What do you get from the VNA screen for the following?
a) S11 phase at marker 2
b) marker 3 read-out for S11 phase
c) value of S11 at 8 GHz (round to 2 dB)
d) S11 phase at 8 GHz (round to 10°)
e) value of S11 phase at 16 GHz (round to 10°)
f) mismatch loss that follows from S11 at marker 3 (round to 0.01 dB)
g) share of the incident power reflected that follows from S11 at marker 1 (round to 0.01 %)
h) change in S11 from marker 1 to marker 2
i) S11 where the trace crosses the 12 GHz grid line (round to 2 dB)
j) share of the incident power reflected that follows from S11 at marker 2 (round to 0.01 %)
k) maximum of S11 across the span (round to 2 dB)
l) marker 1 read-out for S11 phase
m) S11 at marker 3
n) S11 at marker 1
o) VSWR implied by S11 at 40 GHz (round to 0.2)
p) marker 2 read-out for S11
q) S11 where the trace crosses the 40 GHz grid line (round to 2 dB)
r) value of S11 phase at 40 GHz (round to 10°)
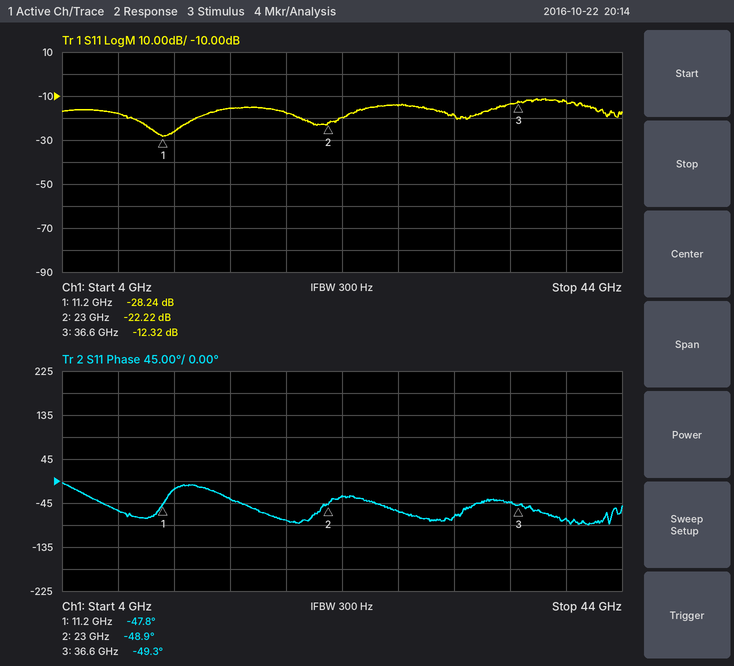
-48.9°
-49.3°
-18 dB
-60°
-40°
0.26 dB
0.15 %
6.02 dB
-26 dB
0.60 %
-12 dB
-47.8°
-12.32 dB
-28.24 dB
1.6
-22.22 dB
-12 dB
-80°
